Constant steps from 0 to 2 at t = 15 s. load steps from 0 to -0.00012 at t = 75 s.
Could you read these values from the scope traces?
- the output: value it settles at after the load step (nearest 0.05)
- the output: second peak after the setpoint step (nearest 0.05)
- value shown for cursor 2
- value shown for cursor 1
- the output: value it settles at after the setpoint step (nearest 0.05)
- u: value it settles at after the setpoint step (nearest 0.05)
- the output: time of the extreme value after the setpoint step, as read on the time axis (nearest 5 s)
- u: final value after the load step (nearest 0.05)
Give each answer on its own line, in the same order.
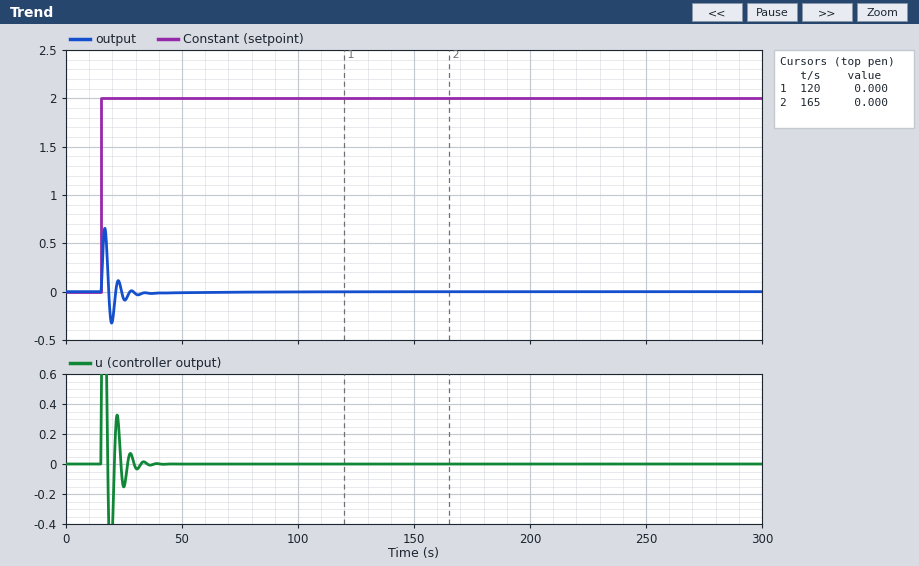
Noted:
0.00
0.10
0.000
0.000
0.00
0.00
15 s
0.00
